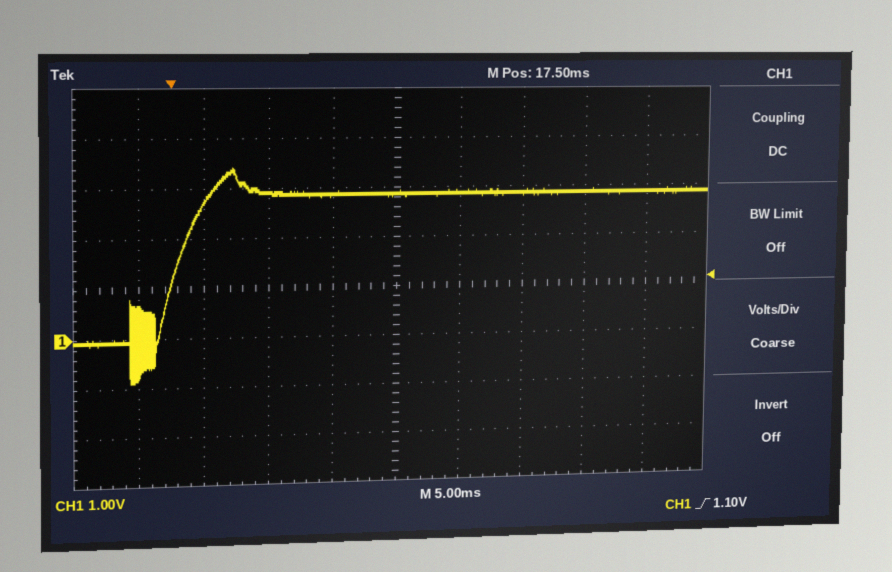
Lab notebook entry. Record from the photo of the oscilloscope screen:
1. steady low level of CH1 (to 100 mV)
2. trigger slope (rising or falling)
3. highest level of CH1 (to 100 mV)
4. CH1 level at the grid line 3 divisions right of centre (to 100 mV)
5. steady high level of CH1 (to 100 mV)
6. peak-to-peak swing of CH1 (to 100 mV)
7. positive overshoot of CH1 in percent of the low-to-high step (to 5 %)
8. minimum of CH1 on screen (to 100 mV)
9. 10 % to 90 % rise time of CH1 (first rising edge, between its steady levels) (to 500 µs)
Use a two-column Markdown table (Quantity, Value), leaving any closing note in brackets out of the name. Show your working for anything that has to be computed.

| Quantity | Value |
|---|---|
| steady low level of CH1 | -100 mV |
| trigger slope | rising |
| highest level of CH1 | 3.4 V |
| CH1 level at the grid line 3 divisions right of centre | 2.9 V |
| steady high level of CH1 | 2.9 V |
| peak-to-peak swing of CH1 | 3.4 V − (-900 mV) = 4.3 V |
| positive overshoot of CH1 in percent of the low-to-high step | 20 % |
| minimum of CH1 on screen | -900 mV |
| 10 % to 90 % rise time of CH1 (first rising edge, between its steady levels) | 3.0 ms |
